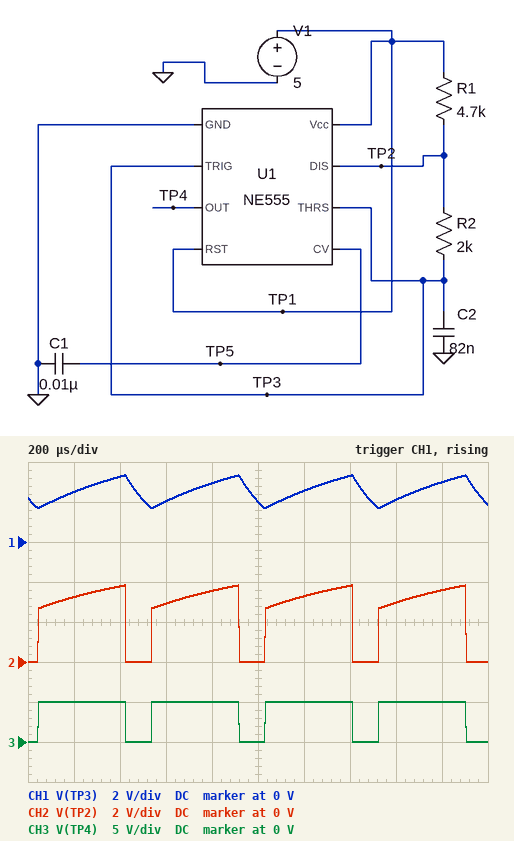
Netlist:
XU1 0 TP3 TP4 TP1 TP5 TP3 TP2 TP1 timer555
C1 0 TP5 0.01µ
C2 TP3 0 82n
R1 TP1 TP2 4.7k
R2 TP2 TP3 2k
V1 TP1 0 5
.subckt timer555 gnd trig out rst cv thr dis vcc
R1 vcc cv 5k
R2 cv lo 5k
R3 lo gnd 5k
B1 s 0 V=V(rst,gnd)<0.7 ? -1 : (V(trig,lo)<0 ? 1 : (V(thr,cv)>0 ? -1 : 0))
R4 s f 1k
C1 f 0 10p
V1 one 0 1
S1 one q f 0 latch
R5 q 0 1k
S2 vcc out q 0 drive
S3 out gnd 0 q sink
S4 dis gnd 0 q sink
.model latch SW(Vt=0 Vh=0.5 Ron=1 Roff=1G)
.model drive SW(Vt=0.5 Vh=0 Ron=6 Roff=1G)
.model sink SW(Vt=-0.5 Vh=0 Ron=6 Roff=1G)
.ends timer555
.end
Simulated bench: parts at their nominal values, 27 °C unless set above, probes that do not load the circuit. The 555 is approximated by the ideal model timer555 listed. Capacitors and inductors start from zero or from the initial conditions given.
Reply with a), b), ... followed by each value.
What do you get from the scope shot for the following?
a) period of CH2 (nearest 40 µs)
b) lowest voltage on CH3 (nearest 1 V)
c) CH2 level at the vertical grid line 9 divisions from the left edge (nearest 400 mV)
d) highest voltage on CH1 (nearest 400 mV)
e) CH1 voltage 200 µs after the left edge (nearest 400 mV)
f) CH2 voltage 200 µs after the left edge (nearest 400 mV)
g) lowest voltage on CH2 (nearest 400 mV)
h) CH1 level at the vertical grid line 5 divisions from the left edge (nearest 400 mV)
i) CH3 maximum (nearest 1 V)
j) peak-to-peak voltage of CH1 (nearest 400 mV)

a) 480 µs
b) 0 V
c) 3.6 V
d) 3.2 V
e) 2.4 V
f) 3.2 V
g) 0 V
h) 2.0 V
i) 5 V
j) 1.6 V
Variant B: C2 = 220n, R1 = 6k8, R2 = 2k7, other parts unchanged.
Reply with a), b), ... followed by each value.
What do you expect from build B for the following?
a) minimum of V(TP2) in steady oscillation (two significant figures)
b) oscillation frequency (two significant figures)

a) 8.1 mV
b) 540 Hz
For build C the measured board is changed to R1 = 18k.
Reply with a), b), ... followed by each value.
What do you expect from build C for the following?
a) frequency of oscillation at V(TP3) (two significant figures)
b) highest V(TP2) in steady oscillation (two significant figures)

a) 800 Hz
b) 3.5 V
